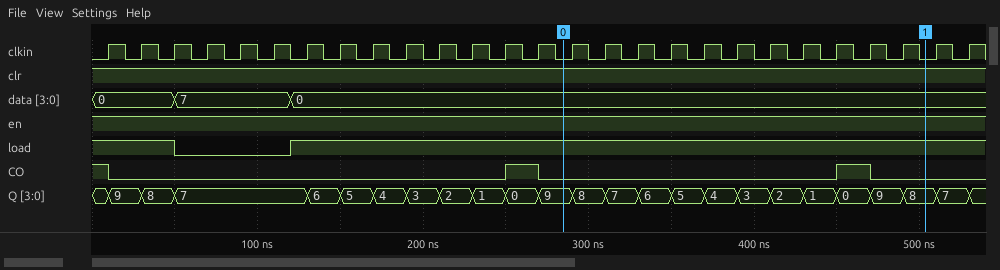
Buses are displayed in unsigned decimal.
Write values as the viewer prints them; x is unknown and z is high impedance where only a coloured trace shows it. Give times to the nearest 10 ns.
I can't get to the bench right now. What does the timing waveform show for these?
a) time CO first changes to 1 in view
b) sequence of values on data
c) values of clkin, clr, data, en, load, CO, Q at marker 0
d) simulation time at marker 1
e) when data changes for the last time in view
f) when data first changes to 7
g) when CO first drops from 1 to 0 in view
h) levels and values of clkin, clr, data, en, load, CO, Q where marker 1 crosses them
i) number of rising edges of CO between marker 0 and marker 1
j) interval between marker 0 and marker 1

250 ns
0, 7, 0
clkin=0, clr=1, data=0, en=1, load=1, CO=0, Q=9
500 ns
120 ns
50 ns
10 ns
clkin=0, clr=1, data=0, en=1, load=1, CO=0, Q=8
1
220 ns
